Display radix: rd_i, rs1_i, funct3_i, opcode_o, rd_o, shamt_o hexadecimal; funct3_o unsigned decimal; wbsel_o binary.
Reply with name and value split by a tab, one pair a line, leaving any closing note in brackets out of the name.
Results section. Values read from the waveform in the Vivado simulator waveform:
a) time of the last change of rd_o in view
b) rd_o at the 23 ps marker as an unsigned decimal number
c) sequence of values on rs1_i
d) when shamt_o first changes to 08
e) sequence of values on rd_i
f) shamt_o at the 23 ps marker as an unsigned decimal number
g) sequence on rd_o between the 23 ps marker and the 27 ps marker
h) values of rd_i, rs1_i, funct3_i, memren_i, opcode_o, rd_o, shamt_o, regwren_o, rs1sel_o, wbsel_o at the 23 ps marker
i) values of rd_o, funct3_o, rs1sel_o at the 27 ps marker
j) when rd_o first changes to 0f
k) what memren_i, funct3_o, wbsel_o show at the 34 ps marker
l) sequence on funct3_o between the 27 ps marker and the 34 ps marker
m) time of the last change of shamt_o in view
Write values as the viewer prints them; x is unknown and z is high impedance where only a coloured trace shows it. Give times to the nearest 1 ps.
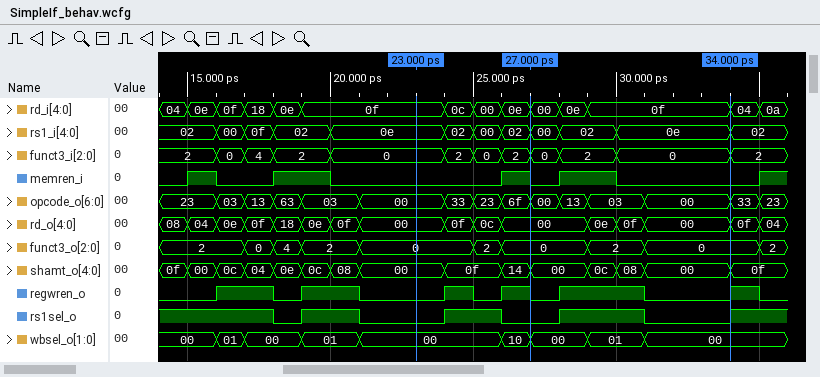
time of the last change of rd_o in view	35 ps
rd_o at the 23 ps marker as an unsigned decimal number	0
sequence of values on rs1_i	02, 00, 0f, 02, 0e, 02, 00, 02, 00, 02, 0e, 02
when shamt_o first changes to 08	20 ps
sequence of values on rd_i	04, 0e, 0f, 18, 0e, 0f, 0c, 00, 0e, 00, 0e, 0f, 04, 0a
shamt_o at the 23 ps marker as an unsigned decimal number	0
sequence on rd_o between the 23 ps marker and the 27 ps marker	00, 0f, 0c, 00
values of rd_i, rs1_i, funct3_i, memren_i, opcode_o, rd_o, shamt_o, regwren_o, rs1sel_o, wbsel_o at the 23 ps marker	rd_i=0f, rs1_i=0e, funct3_i=0, memren_i=0, opcode_o=00, rd_o=00, shamt_o=00, regwren_o=0, rs1sel_o=0, wbsel_o=00
values of rd_o, funct3_o, rs1sel_o at the 27 ps marker	rd_o=00, funct3_o=0, rs1sel_o=0
when rd_o first changes to 0f	17 ps
what memren_i, funct3_o, wbsel_o show at the 34 ps marker	memren_i=0, funct3_o=0, wbsel_o=00
sequence on funct3_o between the 27 ps marker and the 34 ps marker	0, 2, 0
time of the last change of shamt_o in view	34 ps
